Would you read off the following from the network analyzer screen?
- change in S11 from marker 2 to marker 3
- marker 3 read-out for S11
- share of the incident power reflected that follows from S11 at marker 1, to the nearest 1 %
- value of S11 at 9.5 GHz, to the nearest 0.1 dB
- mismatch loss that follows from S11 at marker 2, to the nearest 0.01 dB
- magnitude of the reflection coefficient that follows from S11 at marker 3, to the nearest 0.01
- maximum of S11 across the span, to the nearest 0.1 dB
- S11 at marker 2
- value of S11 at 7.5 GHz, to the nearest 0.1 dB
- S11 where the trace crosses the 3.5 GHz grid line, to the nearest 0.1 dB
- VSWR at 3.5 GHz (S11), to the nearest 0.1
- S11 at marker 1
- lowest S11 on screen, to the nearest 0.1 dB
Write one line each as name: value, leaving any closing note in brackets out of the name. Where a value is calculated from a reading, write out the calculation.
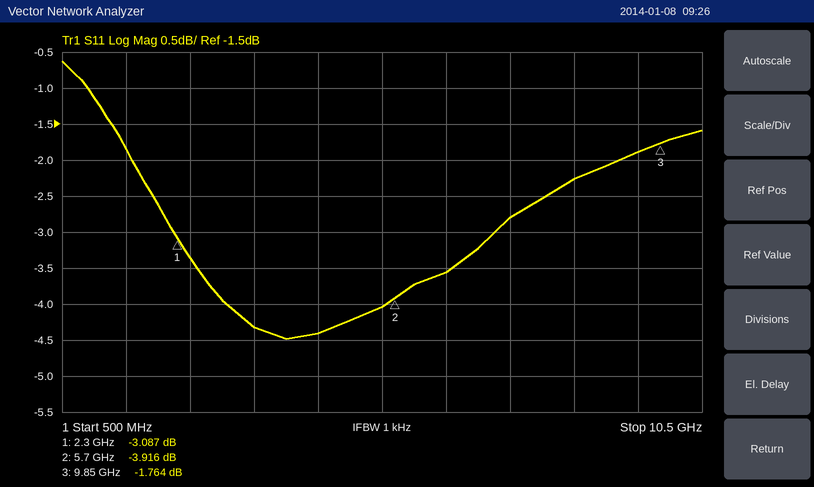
change in S11 from marker 2 to marker 3: -1.764 − (-3.916) = 2.152 dB
marker 3 read-out for S11: -1.764 dB
share of the incident power reflected that follows from S11 at marker 1, to the nearest 1 %: 10^(-3.087/10) ≈ 49 %
value of S11 at 9.5 GHz, to the nearest 0.1 dB: -1.9 dB
mismatch loss that follows from S11 at marker 2, to the nearest 0.01 dB: −10 log10(1 − 10^(-3.916/10)) ≈ 2.26 dB
magnitude of the reflection coefficient that follows from S11 at marker 3, to the nearest 0.01: 10^(-1.764/20) ≈ 0.82
maximum of S11 across the span, to the nearest 0.1 dB: -0.6 dB
S11 at marker 2: -3.916 dB
value of S11 at 7.5 GHz, to the nearest 0.1 dB: -2.8 dB
S11 where the trace crosses the 3.5 GHz grid line, to the nearest 0.1 dB: -4.3 dB
VSWR at 3.5 GHz (S11), to the nearest 0.1: |Γ| = 10^(-4.3/20) = 0.6095; VSWR = (1 + 0.6095)/(1 − 0.6095) ≈ 4.1
S11 at marker 1: -3.087 dB
lowest S11 on screen, to the nearest 0.1 dB: -4.5 dB
